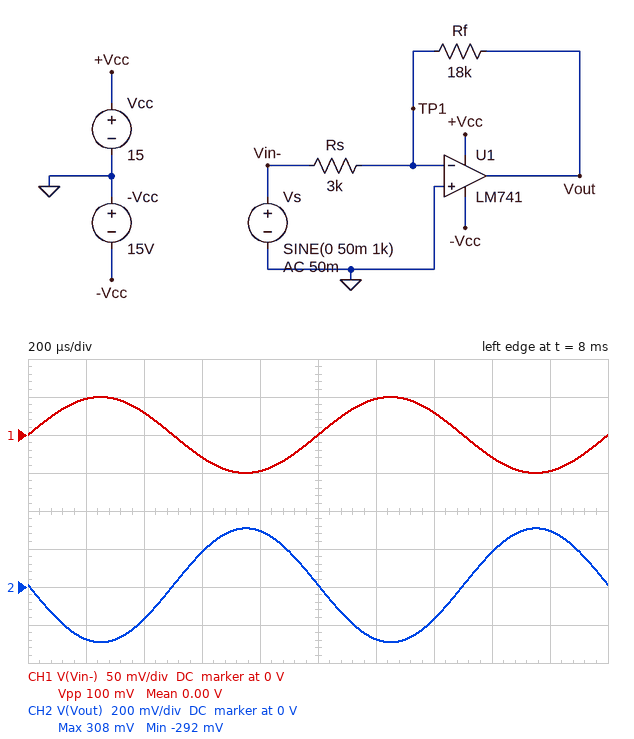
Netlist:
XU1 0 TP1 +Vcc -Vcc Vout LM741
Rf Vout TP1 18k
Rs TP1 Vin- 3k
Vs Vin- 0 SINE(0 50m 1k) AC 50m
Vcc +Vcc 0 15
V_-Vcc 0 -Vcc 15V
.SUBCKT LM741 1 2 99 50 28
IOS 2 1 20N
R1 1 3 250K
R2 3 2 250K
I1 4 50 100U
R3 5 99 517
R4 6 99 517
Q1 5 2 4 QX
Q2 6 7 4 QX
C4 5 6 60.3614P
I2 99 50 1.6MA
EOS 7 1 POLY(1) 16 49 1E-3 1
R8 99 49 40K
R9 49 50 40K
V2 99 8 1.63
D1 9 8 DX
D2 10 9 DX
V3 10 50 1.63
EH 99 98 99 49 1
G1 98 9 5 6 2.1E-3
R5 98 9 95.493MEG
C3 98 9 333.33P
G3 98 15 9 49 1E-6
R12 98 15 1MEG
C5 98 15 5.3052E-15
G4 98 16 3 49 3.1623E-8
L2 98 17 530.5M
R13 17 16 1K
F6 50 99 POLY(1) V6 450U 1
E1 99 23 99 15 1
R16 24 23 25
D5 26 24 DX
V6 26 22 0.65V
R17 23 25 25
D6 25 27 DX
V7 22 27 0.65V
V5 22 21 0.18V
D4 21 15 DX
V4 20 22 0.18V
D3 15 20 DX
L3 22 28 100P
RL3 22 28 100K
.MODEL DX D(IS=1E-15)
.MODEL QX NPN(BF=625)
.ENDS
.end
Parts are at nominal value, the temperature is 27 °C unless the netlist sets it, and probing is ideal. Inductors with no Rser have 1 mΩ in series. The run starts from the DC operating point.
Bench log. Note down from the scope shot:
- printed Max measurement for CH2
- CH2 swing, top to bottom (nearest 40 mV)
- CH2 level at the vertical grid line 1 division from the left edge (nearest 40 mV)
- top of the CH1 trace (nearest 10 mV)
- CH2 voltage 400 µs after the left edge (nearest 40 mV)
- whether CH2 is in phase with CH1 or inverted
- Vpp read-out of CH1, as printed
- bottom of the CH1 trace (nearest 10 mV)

308 mV
600 mV
-280 mV
50 mV
-160 mV
inverted
100 mV
-50 mV
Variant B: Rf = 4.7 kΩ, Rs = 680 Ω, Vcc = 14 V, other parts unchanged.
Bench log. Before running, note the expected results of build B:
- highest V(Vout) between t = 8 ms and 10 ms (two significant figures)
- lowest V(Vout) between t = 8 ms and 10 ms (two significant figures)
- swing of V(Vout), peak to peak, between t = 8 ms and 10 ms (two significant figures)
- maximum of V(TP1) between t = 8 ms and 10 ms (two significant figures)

350 mV
-340 mV
690 mV
1.4 mV
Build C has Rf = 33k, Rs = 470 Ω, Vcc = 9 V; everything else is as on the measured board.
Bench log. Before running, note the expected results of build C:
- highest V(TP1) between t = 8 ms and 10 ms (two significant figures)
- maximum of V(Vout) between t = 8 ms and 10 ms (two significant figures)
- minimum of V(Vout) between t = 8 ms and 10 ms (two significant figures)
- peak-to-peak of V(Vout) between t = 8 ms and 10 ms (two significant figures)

4.6 mV
3.6 V
-3.4 V
7.0 V
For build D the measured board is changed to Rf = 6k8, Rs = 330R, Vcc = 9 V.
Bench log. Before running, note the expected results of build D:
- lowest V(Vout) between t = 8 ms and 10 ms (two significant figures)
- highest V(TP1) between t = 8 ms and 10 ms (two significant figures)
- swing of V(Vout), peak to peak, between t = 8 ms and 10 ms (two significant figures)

-1.0 V
2.1 mV
2.1 V
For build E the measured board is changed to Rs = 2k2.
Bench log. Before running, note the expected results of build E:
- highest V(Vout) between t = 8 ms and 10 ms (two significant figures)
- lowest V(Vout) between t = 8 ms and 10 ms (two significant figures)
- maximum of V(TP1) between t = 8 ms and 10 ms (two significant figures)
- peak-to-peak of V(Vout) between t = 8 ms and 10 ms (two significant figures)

420 mV
-400 mV
1.4 mV
820 mV
